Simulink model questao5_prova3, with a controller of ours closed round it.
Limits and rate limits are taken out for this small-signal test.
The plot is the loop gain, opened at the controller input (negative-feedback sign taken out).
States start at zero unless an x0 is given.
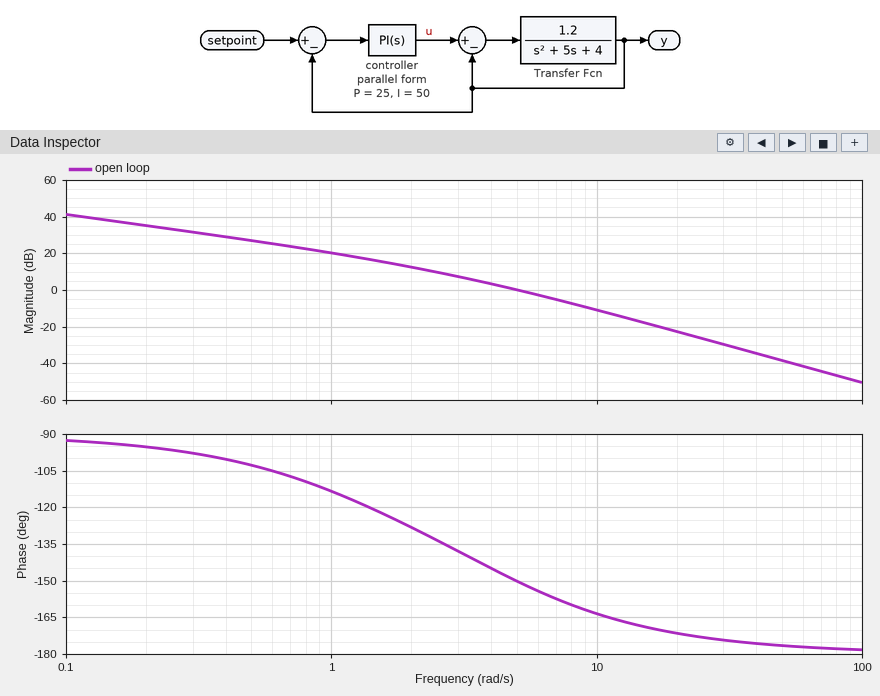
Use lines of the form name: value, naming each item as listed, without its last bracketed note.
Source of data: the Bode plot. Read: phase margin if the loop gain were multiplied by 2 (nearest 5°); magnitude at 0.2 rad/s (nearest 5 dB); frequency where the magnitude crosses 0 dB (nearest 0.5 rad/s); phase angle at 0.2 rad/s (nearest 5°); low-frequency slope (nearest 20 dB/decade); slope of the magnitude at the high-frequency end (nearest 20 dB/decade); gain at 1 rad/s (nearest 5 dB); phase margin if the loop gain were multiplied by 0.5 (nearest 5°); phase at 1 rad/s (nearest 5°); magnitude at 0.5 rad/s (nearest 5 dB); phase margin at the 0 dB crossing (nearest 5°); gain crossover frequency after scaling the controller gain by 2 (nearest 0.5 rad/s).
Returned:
phase margin if the loop gain were multiplied by 2: 20°
magnitude at 0.2 rad/s: 35 dB
frequency where the magnitude crosses 0 dB: 5.0 rad/s
phase angle at 0.2 rad/s: -95°
low-frequency slope: -20 dB/decade
slope of the magnitude at the high-frequency end: -40 dB/decade
gain at 1 rad/s: 20 dB
phase margin if the loop gain were multiplied by 0.5: 40°
phase at 1 rad/s: -115°
magnitude at 0.5 rad/s: 25 dB
phase margin at the 0 dB crossing: 30°
gain crossover frequency after scaling the controller gain by 2: 7.5 rad/s
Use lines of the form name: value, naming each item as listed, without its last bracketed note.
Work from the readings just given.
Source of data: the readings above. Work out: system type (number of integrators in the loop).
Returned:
system type: 1
